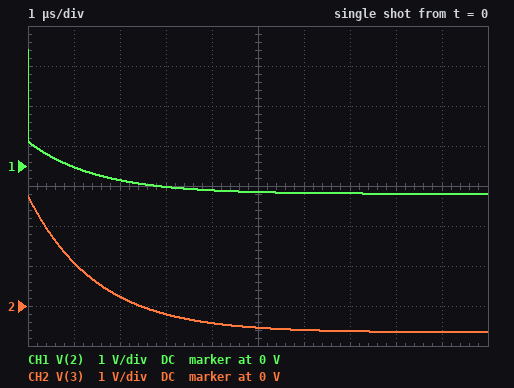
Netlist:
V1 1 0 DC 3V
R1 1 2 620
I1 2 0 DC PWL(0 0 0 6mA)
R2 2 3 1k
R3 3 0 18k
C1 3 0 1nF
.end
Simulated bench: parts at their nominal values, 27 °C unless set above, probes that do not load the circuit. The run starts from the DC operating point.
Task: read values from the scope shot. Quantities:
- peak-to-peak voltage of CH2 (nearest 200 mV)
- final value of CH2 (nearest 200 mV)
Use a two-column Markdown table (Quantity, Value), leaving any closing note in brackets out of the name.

| Quantity | Value |
|---|---|
| peak-to-peak voltage of CH2 | 3.4 V |
| final value of CH2 | -600 mV |
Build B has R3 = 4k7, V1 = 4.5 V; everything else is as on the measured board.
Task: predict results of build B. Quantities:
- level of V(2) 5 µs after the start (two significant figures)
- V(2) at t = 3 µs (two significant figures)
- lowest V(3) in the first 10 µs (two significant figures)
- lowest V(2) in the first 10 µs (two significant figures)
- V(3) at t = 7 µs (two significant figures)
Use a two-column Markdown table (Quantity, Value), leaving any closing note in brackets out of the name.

| Quantity | Value |
|---|---|
| level of V(2) 5 µs after the start | 720 mV |
| V(2) at t = 3 µs | 790 mV |
| lowest V(3) in the first 10 µs | 580 mV |
| lowest V(2) in the first 10 µs | 700 mV |
| V(3) at t = 7 µs | 590 mV |
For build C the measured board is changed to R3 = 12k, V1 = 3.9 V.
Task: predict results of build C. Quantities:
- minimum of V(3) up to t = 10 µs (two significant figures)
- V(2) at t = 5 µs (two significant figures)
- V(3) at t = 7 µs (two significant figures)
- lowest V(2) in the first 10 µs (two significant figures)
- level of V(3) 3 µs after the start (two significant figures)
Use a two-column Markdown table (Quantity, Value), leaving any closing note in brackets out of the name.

| Quantity | Value |
|---|---|
| minimum of V(3) up to t = 10 µs | 160 mV |
| V(2) at t = 5 µs | 210 mV |
| V(3) at t = 7 µs | 180 mV |
| lowest V(2) in the first 10 µs | 170 mV |
| level of V(3) 3 µs after the start | 560 mV |
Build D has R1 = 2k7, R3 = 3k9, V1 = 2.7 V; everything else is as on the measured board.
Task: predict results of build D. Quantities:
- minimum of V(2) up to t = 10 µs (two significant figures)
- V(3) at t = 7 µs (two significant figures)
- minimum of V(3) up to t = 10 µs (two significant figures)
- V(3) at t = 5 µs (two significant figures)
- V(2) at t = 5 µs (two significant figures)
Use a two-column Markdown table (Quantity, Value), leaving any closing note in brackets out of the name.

| Quantity | Value |
|---|---|
| minimum of V(2) up to t = 10 µs | -8.7 V |
| V(3) at t = 7 µs | -6.7 V |
| minimum of V(3) up to t = 10 µs | -6.9 V |
| V(3) at t = 5 µs | -6.3 V |
| V(2) at t = 5 µs | -8.3 V |
